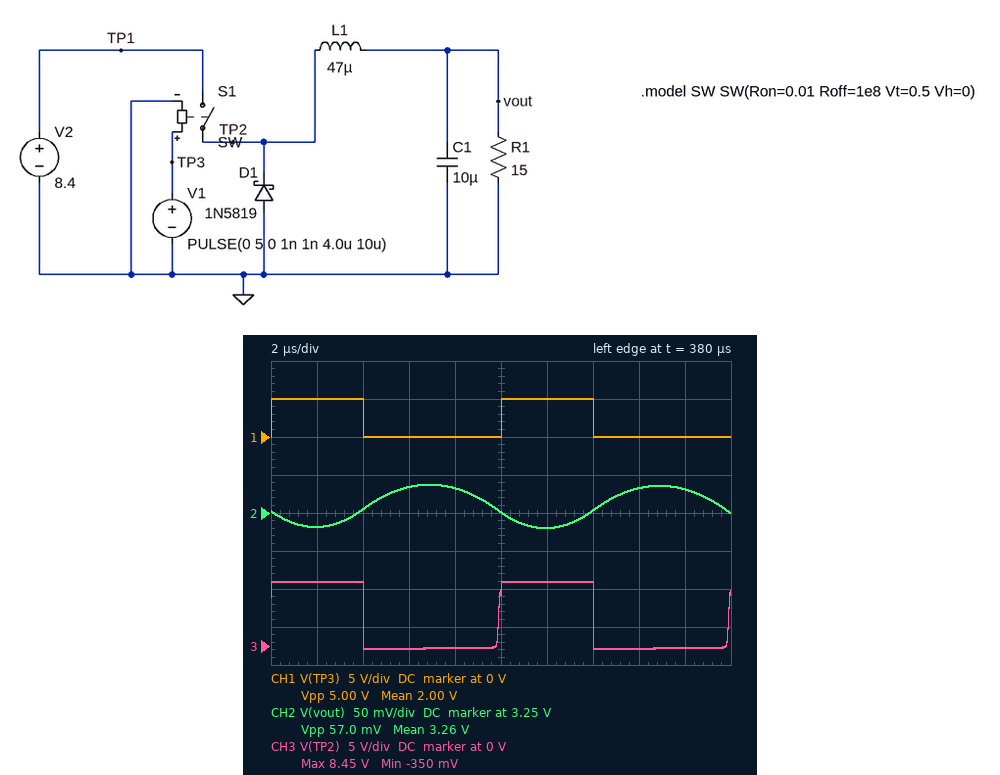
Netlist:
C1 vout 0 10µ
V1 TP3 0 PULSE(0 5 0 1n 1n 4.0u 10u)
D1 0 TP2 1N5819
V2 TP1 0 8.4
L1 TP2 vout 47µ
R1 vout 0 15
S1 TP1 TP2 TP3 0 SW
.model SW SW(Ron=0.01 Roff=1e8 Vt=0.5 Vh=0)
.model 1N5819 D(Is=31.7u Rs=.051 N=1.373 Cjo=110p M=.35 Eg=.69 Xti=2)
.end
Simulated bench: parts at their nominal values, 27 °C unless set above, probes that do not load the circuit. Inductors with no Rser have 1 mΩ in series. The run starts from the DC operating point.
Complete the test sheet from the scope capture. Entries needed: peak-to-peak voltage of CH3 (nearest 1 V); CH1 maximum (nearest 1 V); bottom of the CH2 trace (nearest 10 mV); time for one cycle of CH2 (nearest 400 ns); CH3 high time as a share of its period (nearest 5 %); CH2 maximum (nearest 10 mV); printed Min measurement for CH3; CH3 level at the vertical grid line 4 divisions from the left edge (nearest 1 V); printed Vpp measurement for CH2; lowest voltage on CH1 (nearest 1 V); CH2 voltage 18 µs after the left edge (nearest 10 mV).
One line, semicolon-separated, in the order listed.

9 V; 5 V; 3.23 V; 10.0 µs; 40 %; 3.29 V; -350 mV; 0 V; 57.0 mV; 0 V; 3.28 V
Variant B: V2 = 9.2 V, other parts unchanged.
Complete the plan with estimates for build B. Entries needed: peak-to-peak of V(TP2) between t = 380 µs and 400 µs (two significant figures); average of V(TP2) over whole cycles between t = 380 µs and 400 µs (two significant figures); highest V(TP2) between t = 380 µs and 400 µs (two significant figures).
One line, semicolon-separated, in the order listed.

9.6 V; 3.6 V; 9.2 V
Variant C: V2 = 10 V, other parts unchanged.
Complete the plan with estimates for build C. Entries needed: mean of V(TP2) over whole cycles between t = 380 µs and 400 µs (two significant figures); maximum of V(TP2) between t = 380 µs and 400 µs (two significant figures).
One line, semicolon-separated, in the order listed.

3.9 V; 10 V
